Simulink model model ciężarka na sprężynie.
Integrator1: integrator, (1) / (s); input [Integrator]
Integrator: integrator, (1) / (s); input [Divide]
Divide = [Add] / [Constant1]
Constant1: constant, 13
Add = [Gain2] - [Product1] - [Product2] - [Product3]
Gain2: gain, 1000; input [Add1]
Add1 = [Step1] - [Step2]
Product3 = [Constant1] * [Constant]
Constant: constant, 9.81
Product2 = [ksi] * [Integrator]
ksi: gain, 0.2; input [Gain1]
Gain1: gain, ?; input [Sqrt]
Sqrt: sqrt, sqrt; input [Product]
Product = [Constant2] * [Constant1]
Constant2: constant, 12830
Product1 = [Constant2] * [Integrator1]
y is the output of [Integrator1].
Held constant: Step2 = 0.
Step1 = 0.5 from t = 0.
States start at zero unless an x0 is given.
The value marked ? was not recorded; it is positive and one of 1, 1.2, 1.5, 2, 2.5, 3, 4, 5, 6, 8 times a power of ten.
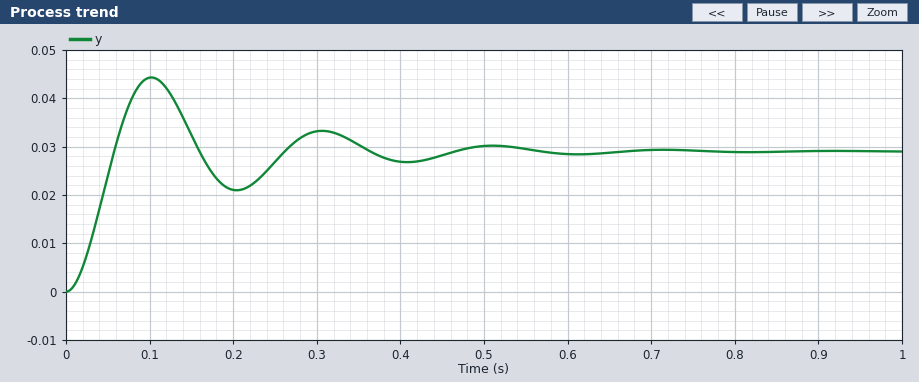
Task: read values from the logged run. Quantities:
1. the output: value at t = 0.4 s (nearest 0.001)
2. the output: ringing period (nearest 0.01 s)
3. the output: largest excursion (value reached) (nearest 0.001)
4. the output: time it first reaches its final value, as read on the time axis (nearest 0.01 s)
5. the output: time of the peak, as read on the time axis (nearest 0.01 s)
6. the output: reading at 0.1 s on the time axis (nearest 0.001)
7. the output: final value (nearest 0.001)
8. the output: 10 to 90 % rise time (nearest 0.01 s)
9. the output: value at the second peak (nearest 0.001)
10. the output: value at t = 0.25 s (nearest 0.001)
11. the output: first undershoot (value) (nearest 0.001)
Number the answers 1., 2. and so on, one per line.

1. 0.027
2. 0.20 s
3. 0.044
4. 0.06 s
5. 0.10 s
6. 0.044
7. 0.029
8. 0.04 s
9. 0.033
10. 0.027
11. 0.021
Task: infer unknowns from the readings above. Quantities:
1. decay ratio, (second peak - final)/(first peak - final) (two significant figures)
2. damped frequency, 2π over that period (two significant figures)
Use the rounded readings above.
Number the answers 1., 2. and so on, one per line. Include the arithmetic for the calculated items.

1. (0.033 - 0.029) / (0.044 - 0.029) = 0.27
2. 2π / 0.2 = 31 rad/s
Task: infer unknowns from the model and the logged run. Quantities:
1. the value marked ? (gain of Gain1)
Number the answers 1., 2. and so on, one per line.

1. 2
